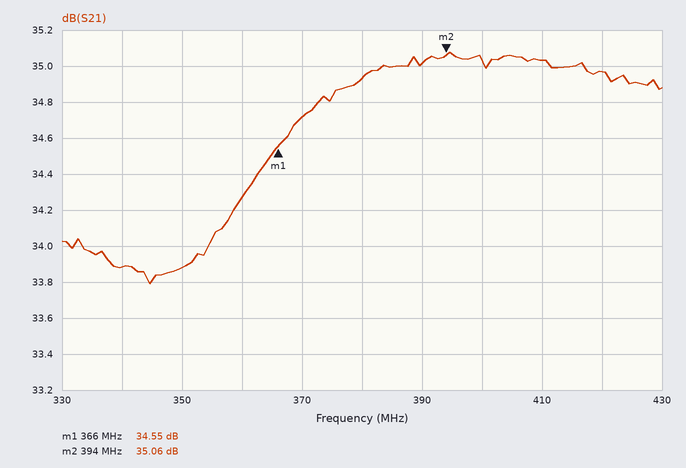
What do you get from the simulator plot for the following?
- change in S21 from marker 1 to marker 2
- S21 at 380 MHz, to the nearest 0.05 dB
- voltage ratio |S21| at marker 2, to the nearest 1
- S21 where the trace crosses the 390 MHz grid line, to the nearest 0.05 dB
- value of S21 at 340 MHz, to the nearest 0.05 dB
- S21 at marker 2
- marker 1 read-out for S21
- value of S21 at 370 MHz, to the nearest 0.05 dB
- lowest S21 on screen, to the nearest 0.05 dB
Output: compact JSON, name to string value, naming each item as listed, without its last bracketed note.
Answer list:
{"change in S21 from marker 1 to marker 2": "0.51 dB", "S21 at 380 MHz, to the nearest 0.05 dB": "34.95 dB", "voltage ratio |S21| at marker 2, to the nearest 1": "57", "S21 where the trace crosses the 390 MHz grid line, to the nearest 0.05 dB": "35.00 dB", "value of S21 at 340 MHz, to the nearest 0.05 dB": "33.90 dB", "S21 at marker 2": "35.06 dB", "marker 1 read-out for S21": "34.55 dB", "value of S21 at 370 MHz, to the nearest 0.05 dB": "34.70 dB", "lowest S21 on screen, to the nearest 0.05 dB": "33.80 dB"}
